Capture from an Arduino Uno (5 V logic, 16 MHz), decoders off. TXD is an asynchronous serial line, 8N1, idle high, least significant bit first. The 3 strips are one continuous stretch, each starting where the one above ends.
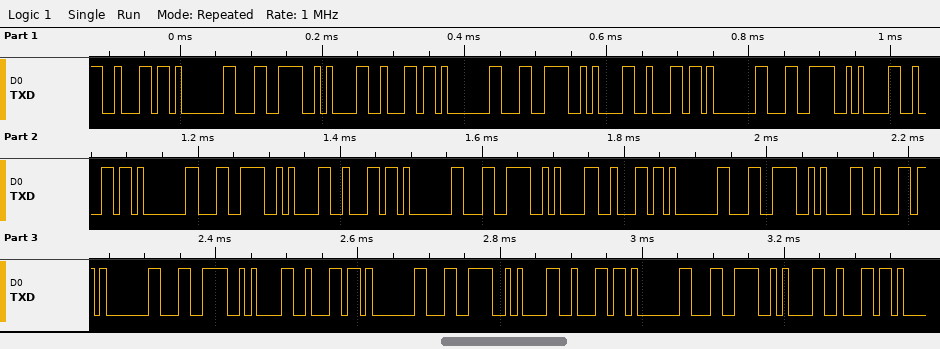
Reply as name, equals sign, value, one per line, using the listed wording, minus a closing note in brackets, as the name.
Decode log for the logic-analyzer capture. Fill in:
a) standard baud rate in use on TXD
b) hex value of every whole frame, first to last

standard baud rate in use on TXD = 115200 baud
hex value of every whole frame, first to last = 62 01 CC 0A 62 01 CC 0A 62 01 CC 0A 62 01 CC 0A 62 01 CC 0A 62 01 CC 0A 62 01 CC 0A 62 01 CC 0A 62 01 CC 0A 62
